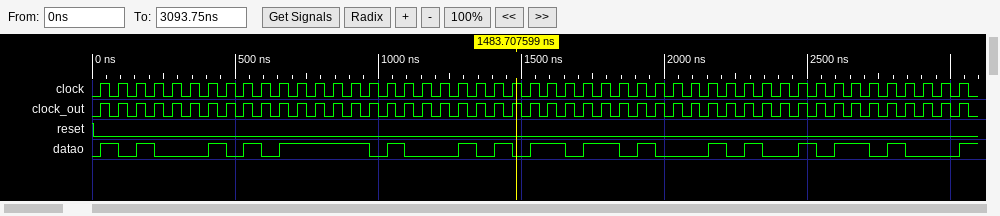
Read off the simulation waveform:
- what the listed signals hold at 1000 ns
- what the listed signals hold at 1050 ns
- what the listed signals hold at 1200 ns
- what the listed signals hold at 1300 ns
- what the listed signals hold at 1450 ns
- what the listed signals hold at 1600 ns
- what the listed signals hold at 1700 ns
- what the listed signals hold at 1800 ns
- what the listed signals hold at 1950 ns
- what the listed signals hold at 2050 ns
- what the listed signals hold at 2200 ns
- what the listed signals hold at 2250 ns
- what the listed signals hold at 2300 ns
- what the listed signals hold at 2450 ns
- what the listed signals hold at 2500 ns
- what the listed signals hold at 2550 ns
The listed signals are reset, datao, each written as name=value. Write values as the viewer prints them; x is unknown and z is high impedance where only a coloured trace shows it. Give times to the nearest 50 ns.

reset=0, datao=0
reset=0, datao=1
reset=0, datao=0
reset=0, datao=1
reset=0, datao=1
reset=0, datao=1
reset=0, datao=0
reset=0, datao=1
reset=0, datao=1
reset=0, datao=0
reset=0, datao=1
reset=0, datao=0
reset=0, datao=1
reset=0, datao=0
reset=0, datao=1
reset=0, datao=0
